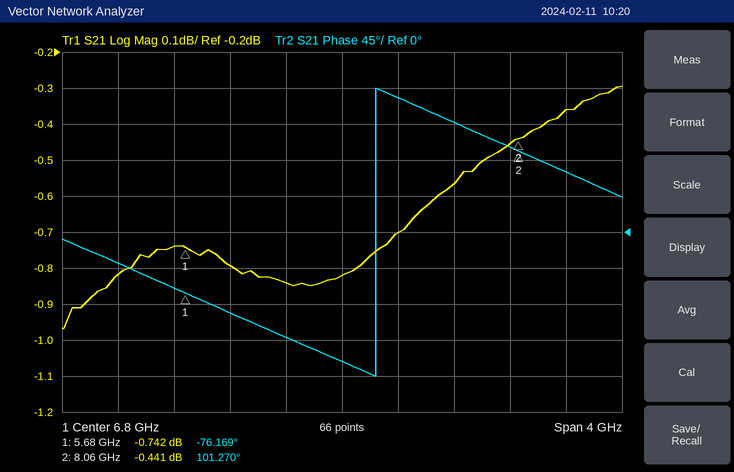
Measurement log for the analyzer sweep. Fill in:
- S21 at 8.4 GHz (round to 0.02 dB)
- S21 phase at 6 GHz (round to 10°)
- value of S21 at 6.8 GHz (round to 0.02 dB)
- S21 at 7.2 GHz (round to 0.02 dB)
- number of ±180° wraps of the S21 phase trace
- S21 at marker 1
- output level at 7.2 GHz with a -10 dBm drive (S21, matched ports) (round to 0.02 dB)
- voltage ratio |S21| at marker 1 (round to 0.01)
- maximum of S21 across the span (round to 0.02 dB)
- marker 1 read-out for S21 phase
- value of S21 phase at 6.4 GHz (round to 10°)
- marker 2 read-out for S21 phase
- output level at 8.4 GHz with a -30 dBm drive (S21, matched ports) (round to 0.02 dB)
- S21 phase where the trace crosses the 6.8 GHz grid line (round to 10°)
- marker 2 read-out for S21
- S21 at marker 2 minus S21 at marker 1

-0.36 dB
-100°
-0.82 dB
-0.70 dB
1
-0.742 dB
-10.70 dBm
0.92
-0.30 dB
-76.169°
-130°
101.270°
-30.36 dBm
-160°
-0.441 dB
0.301 dB
